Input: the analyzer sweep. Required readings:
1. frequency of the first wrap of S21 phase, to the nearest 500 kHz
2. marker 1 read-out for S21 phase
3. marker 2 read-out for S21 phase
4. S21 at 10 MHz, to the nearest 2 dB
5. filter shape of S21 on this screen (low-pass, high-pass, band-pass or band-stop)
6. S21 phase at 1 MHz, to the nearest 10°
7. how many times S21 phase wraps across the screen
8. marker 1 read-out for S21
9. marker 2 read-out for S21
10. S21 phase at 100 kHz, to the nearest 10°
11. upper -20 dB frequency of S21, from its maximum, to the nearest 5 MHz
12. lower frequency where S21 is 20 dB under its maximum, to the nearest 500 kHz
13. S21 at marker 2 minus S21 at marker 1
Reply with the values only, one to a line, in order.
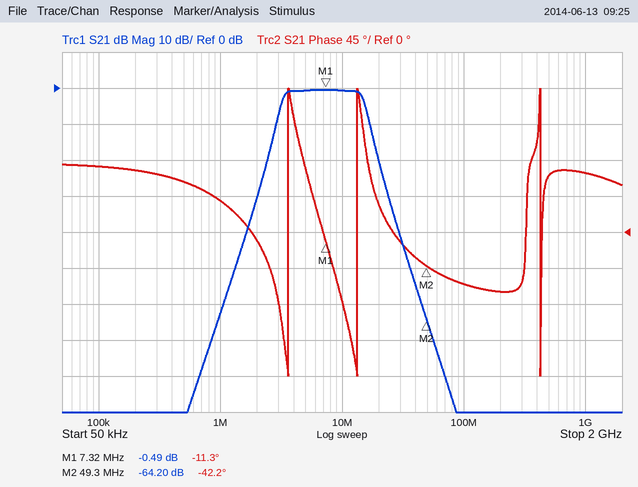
3.5 MHz
-11.3°
-42.2°
0 dB
band-pass
40°
3
-0.49 dB
-64.20 dB
80°
20 MHz
2.5 MHz
-63.71 dB
